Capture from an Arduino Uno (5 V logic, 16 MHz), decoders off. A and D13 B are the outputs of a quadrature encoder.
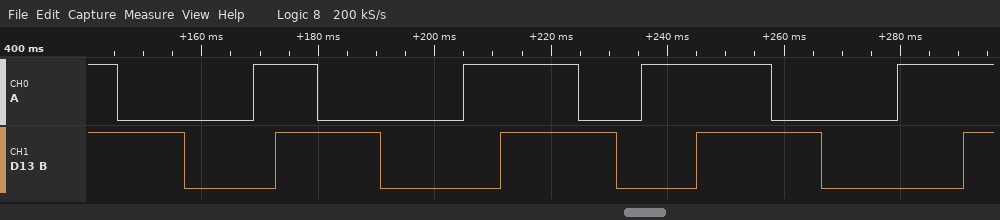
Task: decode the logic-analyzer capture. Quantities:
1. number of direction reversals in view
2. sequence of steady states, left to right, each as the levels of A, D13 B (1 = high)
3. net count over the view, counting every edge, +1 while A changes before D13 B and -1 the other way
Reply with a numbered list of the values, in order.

1. 0
2. 11 01 00 10 11 01 00 10 11 01 00 10 11 01 00 10 11
3. +16
